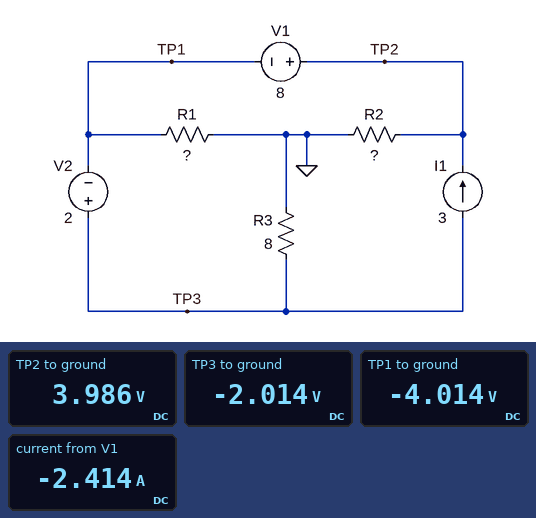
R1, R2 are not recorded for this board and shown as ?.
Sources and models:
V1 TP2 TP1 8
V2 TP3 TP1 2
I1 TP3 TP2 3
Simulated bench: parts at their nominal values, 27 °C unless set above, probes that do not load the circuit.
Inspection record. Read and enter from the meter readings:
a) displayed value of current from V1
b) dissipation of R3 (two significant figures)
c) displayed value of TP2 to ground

-2.414 A
510 mW
3.986 V
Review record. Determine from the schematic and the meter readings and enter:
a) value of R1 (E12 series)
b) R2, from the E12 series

12 Ω
6.8 Ω
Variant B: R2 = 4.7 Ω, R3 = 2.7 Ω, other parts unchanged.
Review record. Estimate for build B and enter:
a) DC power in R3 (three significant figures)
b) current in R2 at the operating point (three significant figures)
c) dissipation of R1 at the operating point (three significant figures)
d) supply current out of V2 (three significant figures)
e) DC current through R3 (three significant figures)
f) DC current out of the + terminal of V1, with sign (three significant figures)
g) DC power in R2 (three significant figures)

1.03 W
922 mA
1.12 W
2.38 A
617 mA
-2.08 A
4.00 W
